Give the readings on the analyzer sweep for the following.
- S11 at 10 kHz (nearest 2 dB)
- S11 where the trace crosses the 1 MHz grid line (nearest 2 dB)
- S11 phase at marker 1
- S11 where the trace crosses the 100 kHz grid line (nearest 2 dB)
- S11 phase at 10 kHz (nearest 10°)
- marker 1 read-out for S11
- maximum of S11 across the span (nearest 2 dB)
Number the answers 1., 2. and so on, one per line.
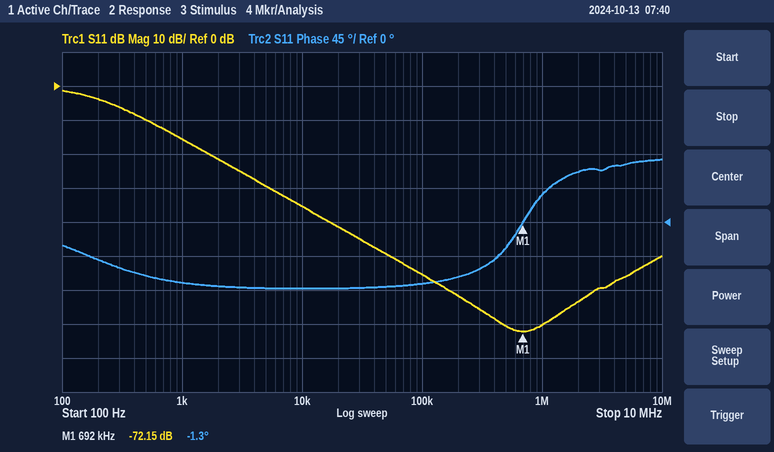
1. -36 dB
2. -70 dB
3. -1.3°
4. -56 dB
5. -90°
6. -72.15 dB
7. -2 dB
